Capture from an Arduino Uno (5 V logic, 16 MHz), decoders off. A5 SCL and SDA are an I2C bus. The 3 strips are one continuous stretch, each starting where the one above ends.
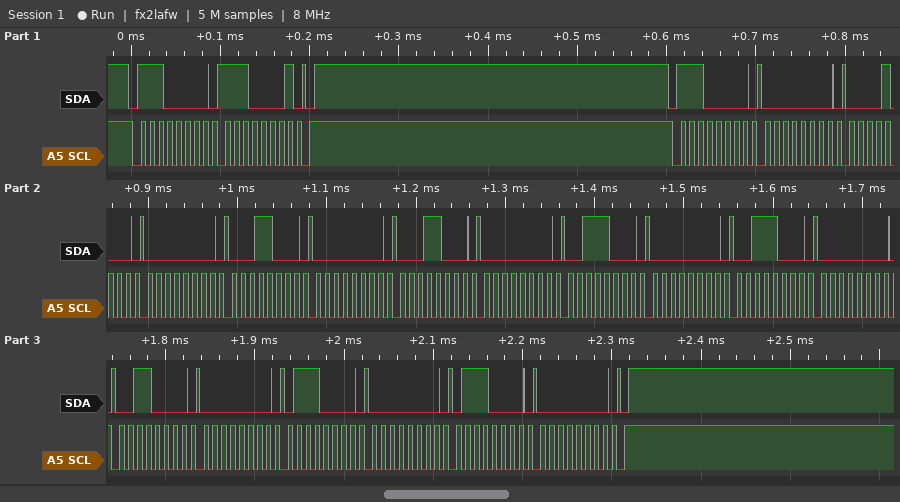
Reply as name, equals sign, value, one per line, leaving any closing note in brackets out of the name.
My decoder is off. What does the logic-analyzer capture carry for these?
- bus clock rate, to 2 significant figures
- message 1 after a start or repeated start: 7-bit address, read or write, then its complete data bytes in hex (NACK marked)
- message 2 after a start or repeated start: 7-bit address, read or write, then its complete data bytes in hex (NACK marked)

bus clock rate, to 2 significant figures = 100 kHz
message 1 after a start or repeated start: 7-bit address, read or write, then its complete data bytes in hex = 0x70 write: E1
message 2 after a start or repeated start: 7-bit address, read or write, then its complete data bytes in hex = 0x70 write: 00 08 00 18 00 18 00 38 00 38 00 30 00 70 00 70 00
